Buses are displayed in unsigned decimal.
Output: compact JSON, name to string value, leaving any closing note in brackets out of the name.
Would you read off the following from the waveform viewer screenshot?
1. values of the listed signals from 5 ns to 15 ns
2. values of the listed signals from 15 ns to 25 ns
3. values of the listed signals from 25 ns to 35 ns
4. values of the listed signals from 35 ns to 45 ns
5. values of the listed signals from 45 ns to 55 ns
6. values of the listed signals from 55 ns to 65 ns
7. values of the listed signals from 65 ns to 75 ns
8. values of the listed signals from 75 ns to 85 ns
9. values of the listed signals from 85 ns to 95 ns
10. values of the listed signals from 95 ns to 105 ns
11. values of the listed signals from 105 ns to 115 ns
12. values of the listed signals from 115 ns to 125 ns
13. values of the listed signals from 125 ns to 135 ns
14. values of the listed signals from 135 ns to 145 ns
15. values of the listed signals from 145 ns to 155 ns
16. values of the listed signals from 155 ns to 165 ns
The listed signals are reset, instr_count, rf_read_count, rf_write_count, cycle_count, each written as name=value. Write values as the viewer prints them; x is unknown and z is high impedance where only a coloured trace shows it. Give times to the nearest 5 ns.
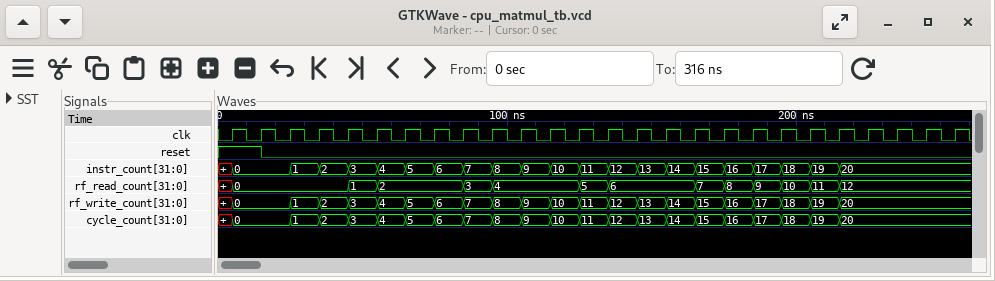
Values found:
{"values of the listed signals from 5 ns to 15 ns": "reset=1, instr_count=0, rf_read_count=0, rf_write_count=0, cycle_count=0", "values of the listed signals from 15 ns to 25 ns": "reset=0, instr_count=0, rf_read_count=0, rf_write_count=0, cycle_count=0", "values of the listed signals from 25 ns to 35 ns": "reset=0, instr_count=1, rf_read_count=0, rf_write_count=1, cycle_count=1", "values of the listed signals from 35 ns to 45 ns": "reset=0, instr_count=2, rf_read_count=0, rf_write_count=2, cycle_count=2", "values of the listed signals from 45 ns to 55 ns": "reset=0, instr_count=3, rf_read_count=1, rf_write_count=3, cycle_count=3", "values of the listed signals from 55 ns to 65 ns": "reset=0, instr_count=4, rf_read_count=2, rf_write_count=4, cycle_count=4", "values of the listed signals from 65 ns to 75 ns": "reset=0, instr_count=5, rf_read_count=2, rf_write_count=5, cycle_count=5", "values of the listed signals from 75 ns to 85 ns": "reset=0, instr_count=6, rf_read_count=2, rf_write_count=6, cycle_count=6", "values of the listed signals from 85 ns to 95 ns": "reset=0, instr_count=7, rf_read_count=3, rf_write_count=7, cycle_count=7", "values of the listed signals from 95 ns to 105 ns": "reset=0, instr_count=8, rf_read_count=4, rf_write_count=8, cycle_count=8", "values of the listed signals from 105 ns to 115 ns": "reset=0, instr_count=9, rf_read_count=4, rf_write_count=9, cycle_count=9", "values of the listed signals from 115 ns to 125 ns": "reset=0, instr_count=10, rf_read_count=4, rf_write_count=10, cycle_count=10", "values of the listed signals from 125 ns to 135 ns": "reset=0, instr_count=11, rf_read_count=5, rf_write_count=11, cycle_count=11", "values of the listed signals from 135 ns to 145 ns": "reset=0, instr_count=12, rf_read_count=6, rf_write_count=12, cycle_count=12", "values of the listed signals from 145 ns to 155 ns": "reset=0, instr_count=13, rf_read_count=6, rf_write_count=13, cycle_count=13", "values of the listed signals from 155 ns to 165 ns": "reset=0, instr_count=14, rf_read_count=6, rf_write_count=14, cycle_count=14"}
